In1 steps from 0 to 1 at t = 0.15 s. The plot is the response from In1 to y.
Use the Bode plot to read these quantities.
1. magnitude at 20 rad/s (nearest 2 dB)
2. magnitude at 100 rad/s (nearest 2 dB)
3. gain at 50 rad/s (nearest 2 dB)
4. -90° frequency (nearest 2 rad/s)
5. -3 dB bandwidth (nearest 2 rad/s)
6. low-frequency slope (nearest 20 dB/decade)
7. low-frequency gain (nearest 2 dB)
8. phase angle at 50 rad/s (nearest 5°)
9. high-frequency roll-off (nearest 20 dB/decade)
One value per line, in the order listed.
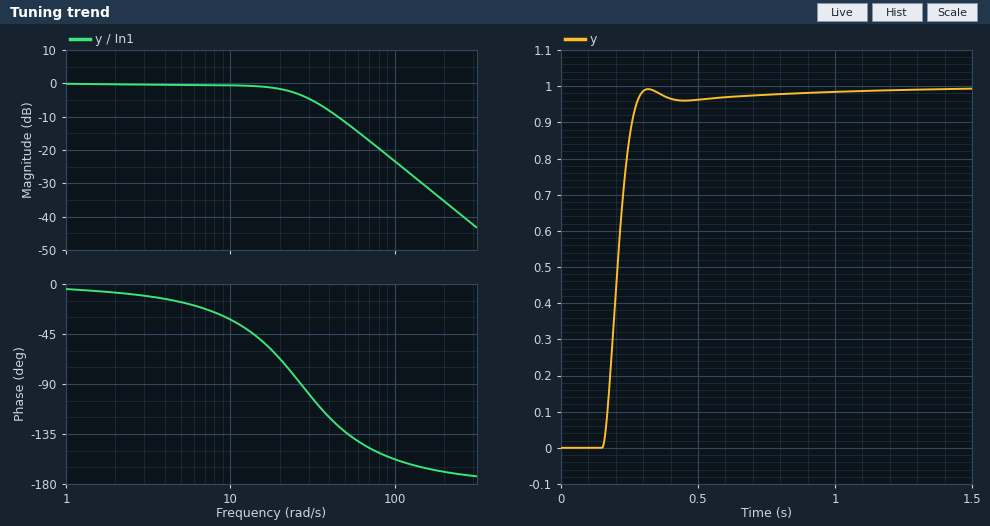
-2 dB
-24 dB
-12 dB
26 rad/s
26 rad/s
0 dB/decade
0 dB
-135°
-40 dB/decade
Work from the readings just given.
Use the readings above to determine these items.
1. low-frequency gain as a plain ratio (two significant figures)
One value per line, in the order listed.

1.0
